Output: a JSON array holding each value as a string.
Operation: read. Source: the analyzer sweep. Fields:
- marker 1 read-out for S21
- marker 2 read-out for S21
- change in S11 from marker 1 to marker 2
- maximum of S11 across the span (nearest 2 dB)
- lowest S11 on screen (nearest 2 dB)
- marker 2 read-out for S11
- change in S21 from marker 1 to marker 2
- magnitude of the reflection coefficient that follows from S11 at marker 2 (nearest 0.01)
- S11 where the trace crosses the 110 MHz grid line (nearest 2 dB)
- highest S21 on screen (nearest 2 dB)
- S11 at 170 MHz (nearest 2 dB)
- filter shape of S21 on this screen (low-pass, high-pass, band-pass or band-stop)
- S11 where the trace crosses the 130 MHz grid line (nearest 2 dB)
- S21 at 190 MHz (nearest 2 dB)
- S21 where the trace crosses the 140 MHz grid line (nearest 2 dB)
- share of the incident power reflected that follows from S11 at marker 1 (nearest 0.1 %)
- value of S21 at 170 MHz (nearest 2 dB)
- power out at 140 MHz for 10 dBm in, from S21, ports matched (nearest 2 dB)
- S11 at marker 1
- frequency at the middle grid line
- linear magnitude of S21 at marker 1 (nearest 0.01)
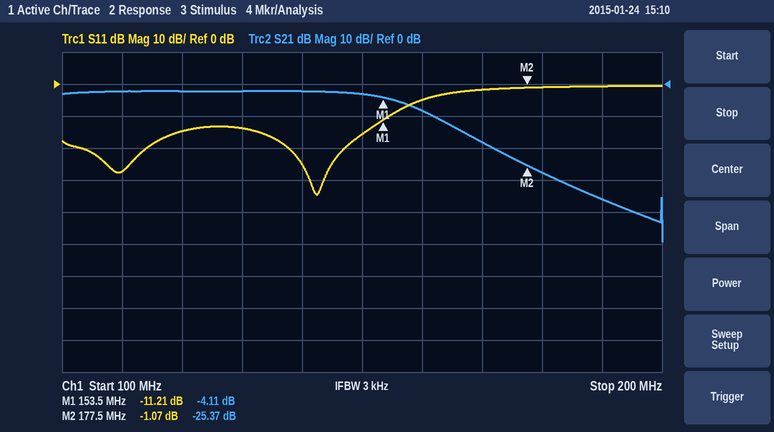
["-4.11 dB", "-25.37 dB", "10.14 dB", "0 dB", "-34 dB", "-1.07 dB", "-21.26 dB", "0.88", "-28 dB", "-2 dB", "-2 dB", "low-pass", "-14 dB", "-36 dB", "-2 dB", "7.6 %", "-18 dB", "8 dBm", "-11.21 dB", "150 MHz", "0.62"]
